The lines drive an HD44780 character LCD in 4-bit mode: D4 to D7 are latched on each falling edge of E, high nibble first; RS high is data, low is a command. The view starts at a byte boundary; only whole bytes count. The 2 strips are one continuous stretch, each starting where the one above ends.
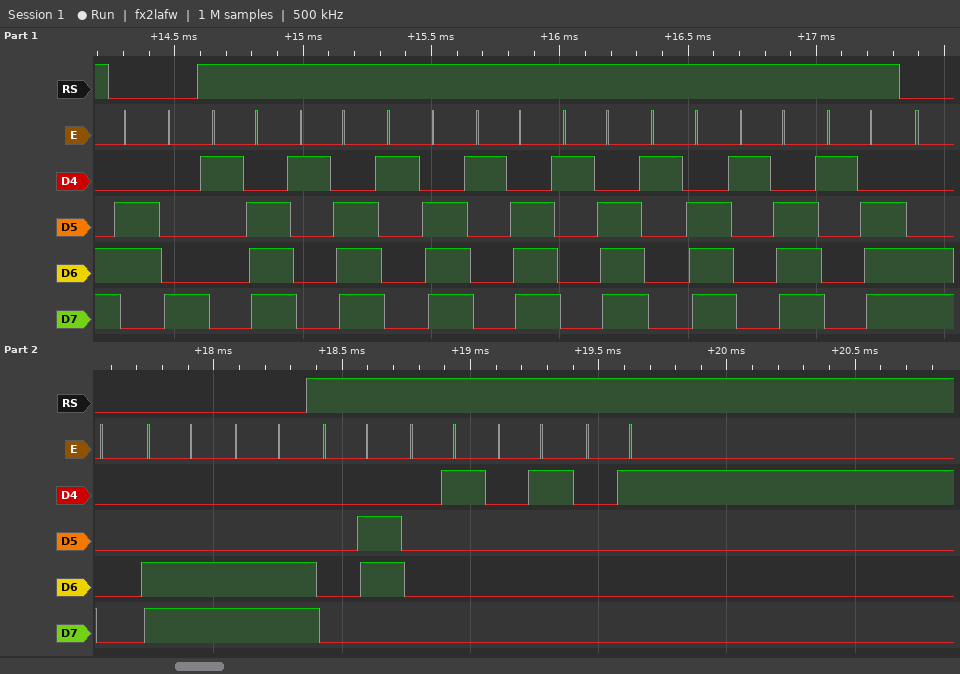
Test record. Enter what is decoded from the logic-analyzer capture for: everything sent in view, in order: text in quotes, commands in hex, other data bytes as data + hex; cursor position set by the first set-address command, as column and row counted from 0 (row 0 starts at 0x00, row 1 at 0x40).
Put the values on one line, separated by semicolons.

0x68 data 1E 1E 1E 1E 1E 1E 1E 1E 0xC0 0xCC 0xCC data 06 01 01 01; column 0, row 1
